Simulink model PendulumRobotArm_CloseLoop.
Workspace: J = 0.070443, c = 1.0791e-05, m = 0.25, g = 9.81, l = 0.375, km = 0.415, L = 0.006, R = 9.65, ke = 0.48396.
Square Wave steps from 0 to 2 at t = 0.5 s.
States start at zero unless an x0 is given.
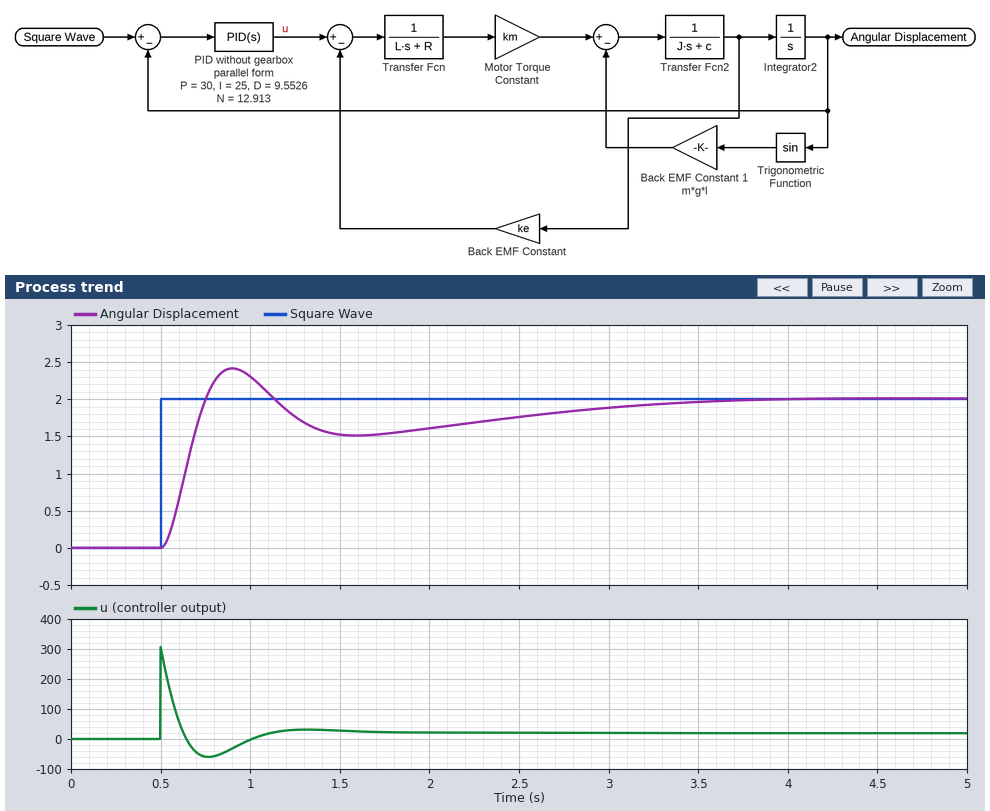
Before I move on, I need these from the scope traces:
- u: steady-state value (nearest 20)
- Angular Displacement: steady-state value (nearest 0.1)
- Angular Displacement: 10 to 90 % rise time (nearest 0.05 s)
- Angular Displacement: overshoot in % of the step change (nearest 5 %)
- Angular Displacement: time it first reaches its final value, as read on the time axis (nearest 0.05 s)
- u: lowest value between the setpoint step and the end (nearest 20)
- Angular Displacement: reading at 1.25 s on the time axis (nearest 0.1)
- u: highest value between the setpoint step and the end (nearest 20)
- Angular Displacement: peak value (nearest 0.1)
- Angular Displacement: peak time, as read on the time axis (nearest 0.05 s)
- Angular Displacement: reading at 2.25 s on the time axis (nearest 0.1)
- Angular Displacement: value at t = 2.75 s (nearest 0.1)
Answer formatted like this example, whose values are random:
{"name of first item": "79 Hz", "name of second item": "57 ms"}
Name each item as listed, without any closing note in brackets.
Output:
{"u: steady-state value": "20", "Angular Displacement: steady-state value": "2.0", "Angular Displacement: 10 to 90 % rise time": "0.15 s", "Angular Displacement: overshoot in % of the step change": "20 %", "Angular Displacement: time it first reaches its final value, as read on the time axis": "0.75 s", "u: lowest value between the setpoint step and the end": "-60", "Angular Displacement: reading at 1.25 s on the time axis": "1.8", "u: highest value between the setpoint step and the end": "300", "Angular Displacement: peak value": "2.4", "Angular Displacement: peak time, as read on the time axis": "0.90 s", "Angular Displacement: reading at 2.25 s on the time axis": "1.7", "Angular Displacement: value at t = 2.75 s": "1.8"}
